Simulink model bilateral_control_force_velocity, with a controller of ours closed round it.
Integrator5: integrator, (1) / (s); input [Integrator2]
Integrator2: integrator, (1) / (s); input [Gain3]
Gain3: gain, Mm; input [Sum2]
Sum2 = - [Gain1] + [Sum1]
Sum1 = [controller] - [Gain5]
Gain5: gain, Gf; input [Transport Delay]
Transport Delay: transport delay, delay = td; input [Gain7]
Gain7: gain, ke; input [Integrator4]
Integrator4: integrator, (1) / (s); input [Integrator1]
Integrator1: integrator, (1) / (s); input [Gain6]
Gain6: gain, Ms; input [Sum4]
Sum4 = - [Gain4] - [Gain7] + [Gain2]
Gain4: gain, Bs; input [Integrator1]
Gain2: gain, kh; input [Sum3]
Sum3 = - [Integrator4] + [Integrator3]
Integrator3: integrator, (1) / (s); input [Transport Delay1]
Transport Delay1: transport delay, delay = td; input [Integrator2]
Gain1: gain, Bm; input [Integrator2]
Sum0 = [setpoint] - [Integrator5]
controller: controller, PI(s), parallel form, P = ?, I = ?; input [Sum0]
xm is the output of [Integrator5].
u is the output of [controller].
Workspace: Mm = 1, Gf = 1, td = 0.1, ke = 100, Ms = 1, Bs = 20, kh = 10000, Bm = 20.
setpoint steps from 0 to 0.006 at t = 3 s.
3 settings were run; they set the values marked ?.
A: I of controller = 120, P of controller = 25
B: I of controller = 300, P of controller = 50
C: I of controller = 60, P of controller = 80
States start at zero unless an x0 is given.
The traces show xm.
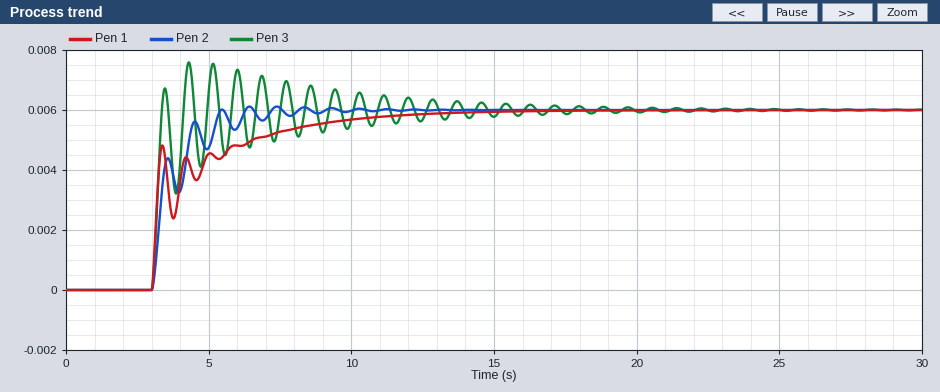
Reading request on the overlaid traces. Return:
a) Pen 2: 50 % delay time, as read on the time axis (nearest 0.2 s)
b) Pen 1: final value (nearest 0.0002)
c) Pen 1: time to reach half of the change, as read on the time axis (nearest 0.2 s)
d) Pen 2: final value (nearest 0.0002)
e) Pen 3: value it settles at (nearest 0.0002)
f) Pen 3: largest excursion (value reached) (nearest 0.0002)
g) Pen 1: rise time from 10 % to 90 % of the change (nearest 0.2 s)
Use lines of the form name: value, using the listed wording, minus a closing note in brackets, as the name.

Pen 2: 50 % delay time, as read on the time axis: 3.4 s
Pen 1: final value: 0.0060
Pen 1: time to reach half of the change, as read on the time axis: 3.2 s
Pen 2: final value: 0.0060
Pen 3: value it settles at: 0.0060
Pen 3: largest excursion (value reached): 0.0076
Pen 1: rise time from 10 % to 90 % of the change: 5.0 s
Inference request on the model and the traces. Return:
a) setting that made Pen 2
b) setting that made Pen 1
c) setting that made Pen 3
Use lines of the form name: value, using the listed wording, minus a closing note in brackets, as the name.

setting that made Pen 2: A
setting that made Pen 1: C
setting that made Pen 3: B
